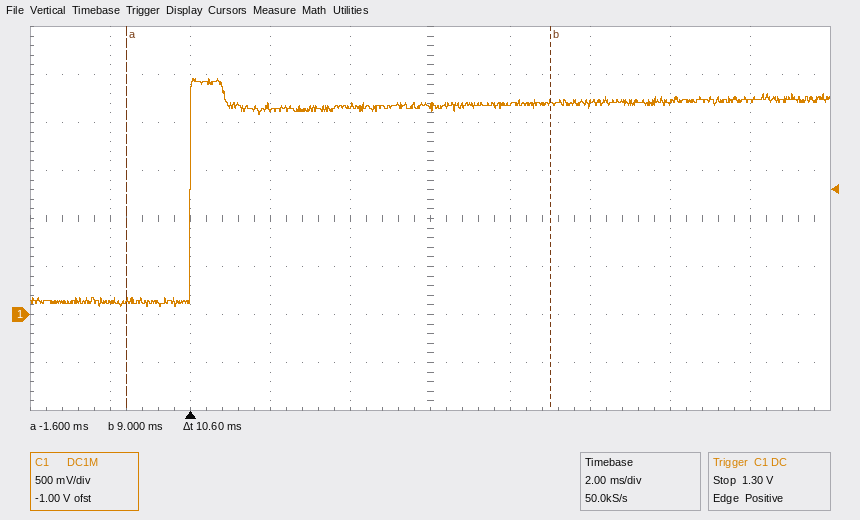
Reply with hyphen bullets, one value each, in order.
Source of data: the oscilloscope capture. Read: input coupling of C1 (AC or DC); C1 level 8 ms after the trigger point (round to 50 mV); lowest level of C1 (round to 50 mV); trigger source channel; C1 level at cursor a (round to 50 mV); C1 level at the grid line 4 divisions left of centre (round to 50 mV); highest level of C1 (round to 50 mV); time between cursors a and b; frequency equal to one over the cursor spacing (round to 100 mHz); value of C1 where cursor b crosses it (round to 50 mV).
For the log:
- DC
- 2.20 V
- 100 mV
- C1
- 150 mV
- 150 mV
- 2.45 V
- 10.6 ms
- 94.3 Hz
- 2.20 V
